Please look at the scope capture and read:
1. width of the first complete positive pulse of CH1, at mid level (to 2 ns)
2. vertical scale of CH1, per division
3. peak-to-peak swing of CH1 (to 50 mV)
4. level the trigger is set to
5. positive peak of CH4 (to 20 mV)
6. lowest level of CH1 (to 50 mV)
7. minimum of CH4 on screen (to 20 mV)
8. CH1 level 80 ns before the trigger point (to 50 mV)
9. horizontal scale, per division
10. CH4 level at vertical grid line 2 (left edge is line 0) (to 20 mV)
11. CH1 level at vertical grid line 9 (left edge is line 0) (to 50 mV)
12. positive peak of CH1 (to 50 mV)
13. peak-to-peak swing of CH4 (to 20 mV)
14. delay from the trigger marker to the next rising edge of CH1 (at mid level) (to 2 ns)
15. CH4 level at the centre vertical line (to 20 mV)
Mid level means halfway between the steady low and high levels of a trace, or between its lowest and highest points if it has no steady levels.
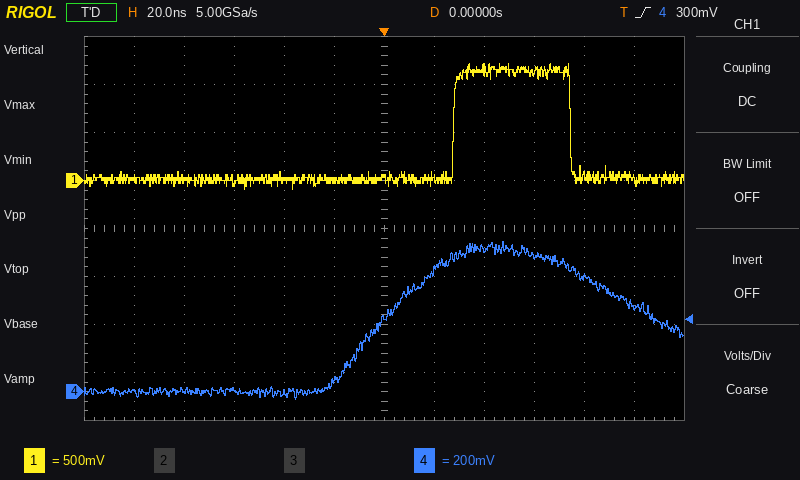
46 ns
500 mV
1.30 V
300 mV
620 mV
-100 mV
-40 mV
0 mV
20 ns
0 mV
1.15 V
1.20 V
660 mV
28 ns
300 mV
